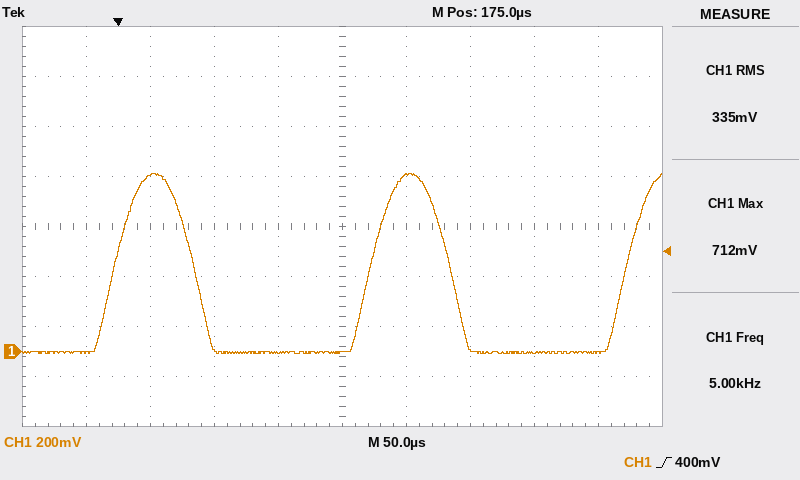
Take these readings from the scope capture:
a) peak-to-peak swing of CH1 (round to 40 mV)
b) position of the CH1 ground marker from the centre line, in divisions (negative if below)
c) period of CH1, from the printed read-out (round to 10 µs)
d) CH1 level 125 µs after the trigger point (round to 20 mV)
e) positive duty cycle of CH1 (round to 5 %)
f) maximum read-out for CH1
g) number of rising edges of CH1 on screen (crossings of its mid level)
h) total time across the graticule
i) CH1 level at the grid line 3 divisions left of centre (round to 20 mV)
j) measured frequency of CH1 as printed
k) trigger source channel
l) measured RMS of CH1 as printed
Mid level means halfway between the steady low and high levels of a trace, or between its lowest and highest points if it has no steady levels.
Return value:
720 mV
-2.5 div
200 µs
0 mV
30 %
712 mV
3
500 µs
700 mV
5.00 kHz
CH1
335 mV
